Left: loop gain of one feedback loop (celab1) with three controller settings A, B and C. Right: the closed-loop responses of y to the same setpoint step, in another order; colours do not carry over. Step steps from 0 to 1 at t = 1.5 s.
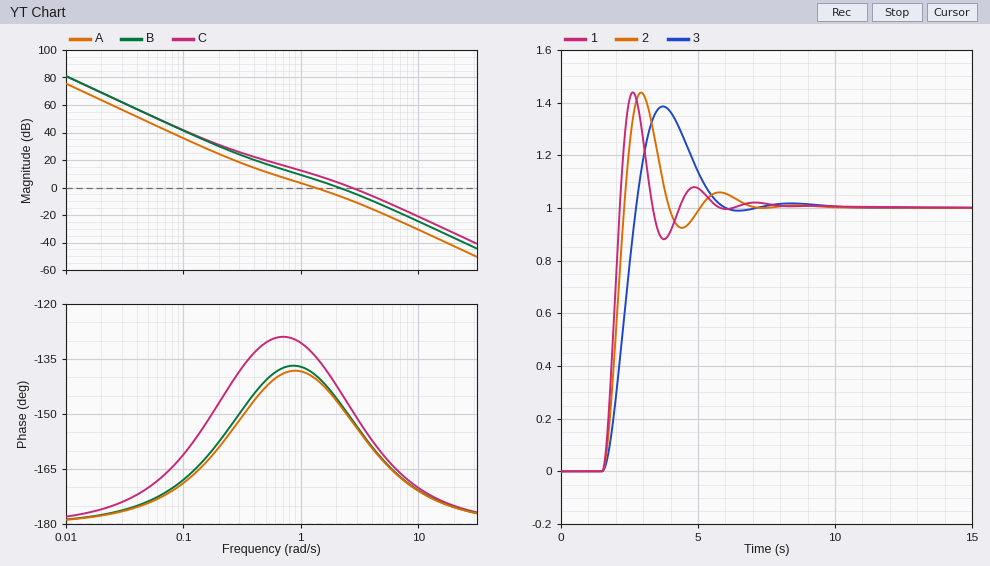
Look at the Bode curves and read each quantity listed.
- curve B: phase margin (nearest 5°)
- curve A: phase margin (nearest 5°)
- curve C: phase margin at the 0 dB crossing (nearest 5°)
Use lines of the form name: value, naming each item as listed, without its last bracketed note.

curve B: phase margin: 35°
curve A: phase margin: 40°
curve C: phase margin at the 0 dB crossing: 30°
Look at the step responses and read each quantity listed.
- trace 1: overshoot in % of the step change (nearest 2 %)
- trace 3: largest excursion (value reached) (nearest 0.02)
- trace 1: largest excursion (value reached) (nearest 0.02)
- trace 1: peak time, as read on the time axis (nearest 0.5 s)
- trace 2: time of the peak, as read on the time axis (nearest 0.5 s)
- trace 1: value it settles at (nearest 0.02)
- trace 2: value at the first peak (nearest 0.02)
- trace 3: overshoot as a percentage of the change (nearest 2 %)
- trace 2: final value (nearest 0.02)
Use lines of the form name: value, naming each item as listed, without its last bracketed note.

trace 1: overshoot in % of the step change: 44 %
trace 3: largest excursion (value reached): 1.38
trace 1: largest excursion (value reached): 1.44
trace 1: peak time, as read on the time axis: 2.5 s
trace 2: time of the peak, as read on the time axis: 3.0 s
trace 1: value it settles at: 1.00
trace 2: value at the first peak: 1.44
trace 3: overshoot as a percentage of the change: 38 %
trace 2: final value: 1.00
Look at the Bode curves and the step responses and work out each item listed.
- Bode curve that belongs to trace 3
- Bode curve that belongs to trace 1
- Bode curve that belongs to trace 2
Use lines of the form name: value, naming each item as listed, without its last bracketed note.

Bode curve that belongs to trace 3: A
Bode curve that belongs to trace 1: C
Bode curve that belongs to trace 2: B
